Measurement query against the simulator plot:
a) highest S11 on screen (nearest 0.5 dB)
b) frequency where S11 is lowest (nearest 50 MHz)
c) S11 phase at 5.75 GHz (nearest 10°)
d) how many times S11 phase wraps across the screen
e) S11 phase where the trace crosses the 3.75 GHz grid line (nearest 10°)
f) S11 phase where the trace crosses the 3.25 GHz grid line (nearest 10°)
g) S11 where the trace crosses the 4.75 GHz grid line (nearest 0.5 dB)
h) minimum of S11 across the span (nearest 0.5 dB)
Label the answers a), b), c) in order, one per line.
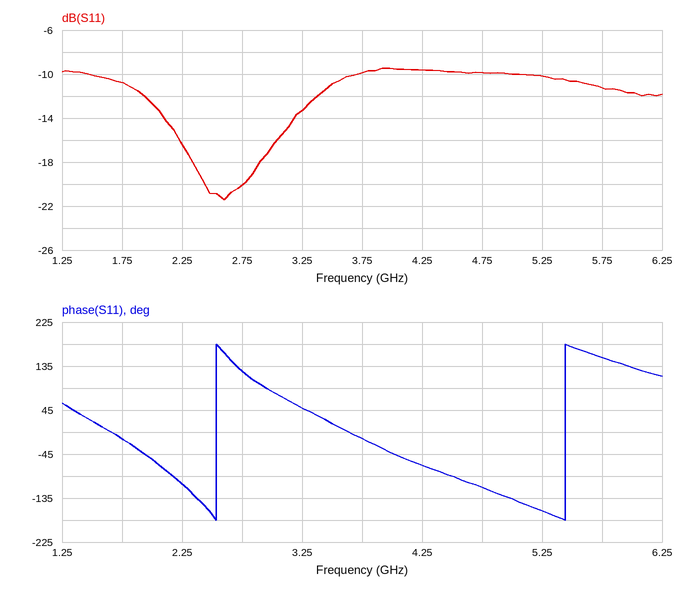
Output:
a) -9.5 dB
b) 2.60 GHz
c) 150°
d) 2
e) -10°
f) 50°
g) -10.0 dB
h) -21.5 dB
